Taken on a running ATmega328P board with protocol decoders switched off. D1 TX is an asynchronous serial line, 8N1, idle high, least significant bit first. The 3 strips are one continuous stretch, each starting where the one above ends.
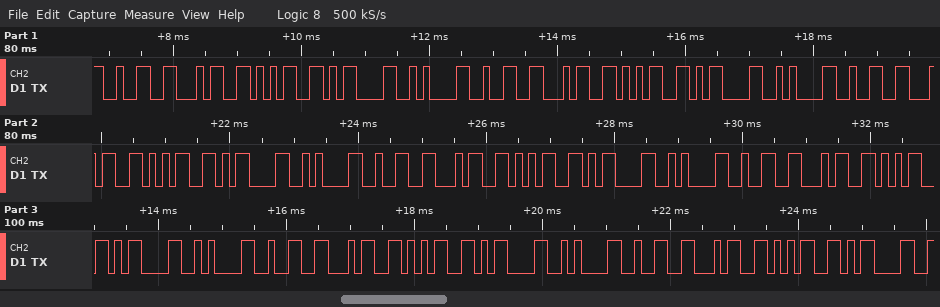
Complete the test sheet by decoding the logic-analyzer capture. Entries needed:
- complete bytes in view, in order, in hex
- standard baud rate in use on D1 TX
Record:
32 34 35 0D 0A 32 34 35 0D 0A 32 34 35 0D 0A 32 34 35 0D 0A 32 34 35 0D 0A 32 34 35 0D 0A 32 34 35 0D
9600 baud
